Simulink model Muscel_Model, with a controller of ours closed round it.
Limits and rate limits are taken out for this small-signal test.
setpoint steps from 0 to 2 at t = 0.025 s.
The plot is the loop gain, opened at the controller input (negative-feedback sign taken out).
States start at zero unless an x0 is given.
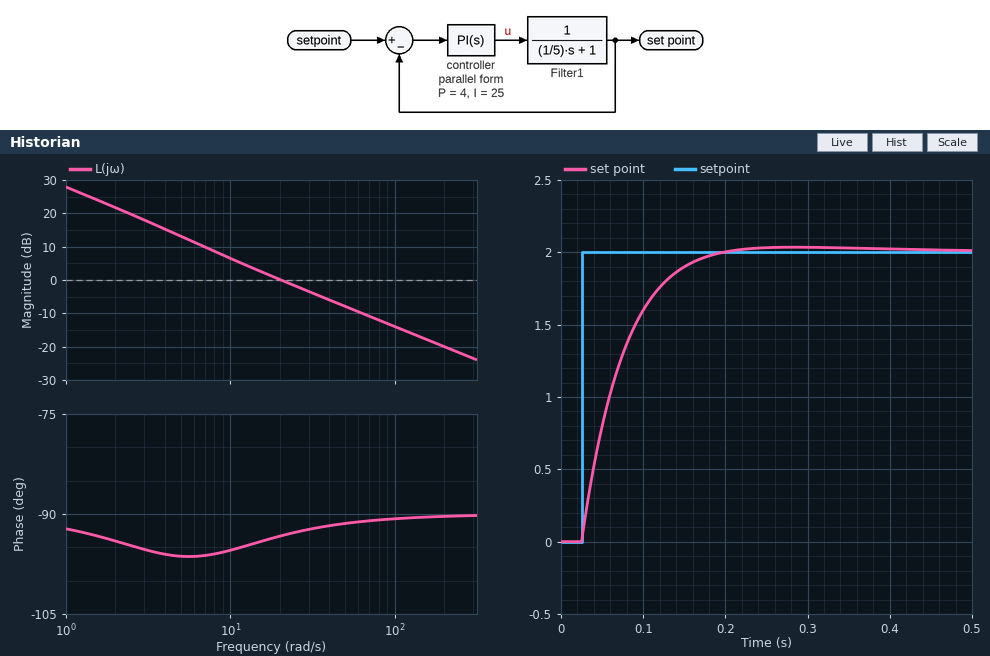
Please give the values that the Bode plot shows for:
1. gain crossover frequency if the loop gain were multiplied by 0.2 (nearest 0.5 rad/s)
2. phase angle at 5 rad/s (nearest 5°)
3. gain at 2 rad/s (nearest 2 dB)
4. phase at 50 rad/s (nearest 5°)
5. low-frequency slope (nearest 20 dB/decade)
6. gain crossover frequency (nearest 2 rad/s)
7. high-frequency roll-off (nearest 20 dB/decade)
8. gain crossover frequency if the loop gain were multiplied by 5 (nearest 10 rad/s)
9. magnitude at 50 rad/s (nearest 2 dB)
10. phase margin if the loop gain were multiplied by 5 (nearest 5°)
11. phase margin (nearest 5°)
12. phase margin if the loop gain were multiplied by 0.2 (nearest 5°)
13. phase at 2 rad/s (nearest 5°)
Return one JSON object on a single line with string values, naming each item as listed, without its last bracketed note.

{"gain crossover frequency if the loop gain were multiplied by 0.2": "4.5 rad/s", "phase angle at 5 rad/s": "-95°", "gain at 2 rad/s": "22 dB", "phase at 50 rad/s": "-90°", "low-frequency slope": "-20 dB/decade", "gain crossover frequency": "20 rad/s", "high-frequency roll-off": "-20 dB/decade", "gain crossover frequency if the loop gain were multiplied by 5": "100 rad/s", "magnitude at 50 rad/s": "-8 dB", "phase margin if the loop gain were multiplied by 5": "90°", "phase margin": "85°", "phase margin if the loop gain were multiplied by 0.2": "85°", "phase at 2 rad/s": "-95°"}
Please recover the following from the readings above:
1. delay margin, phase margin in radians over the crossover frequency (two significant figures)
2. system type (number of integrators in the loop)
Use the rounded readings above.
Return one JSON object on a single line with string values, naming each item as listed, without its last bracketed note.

{"delay margin, phase margin in radians over the crossover frequency": "0.074 s", "system type": "1"}
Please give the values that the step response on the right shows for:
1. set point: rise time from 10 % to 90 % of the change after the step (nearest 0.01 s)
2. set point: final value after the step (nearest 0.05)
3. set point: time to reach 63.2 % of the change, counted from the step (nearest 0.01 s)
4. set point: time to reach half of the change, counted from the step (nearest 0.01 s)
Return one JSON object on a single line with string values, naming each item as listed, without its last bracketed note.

{"set point: rise time from 10 % to 90 % of the change after the step": "0.10 s", "set point: final value after the step": "2.00", "set point: time to reach 63.2 % of the change, counted from the step": "0.05 s", "set point: time to reach half of the change, counted from the step": "0.03 s"}
